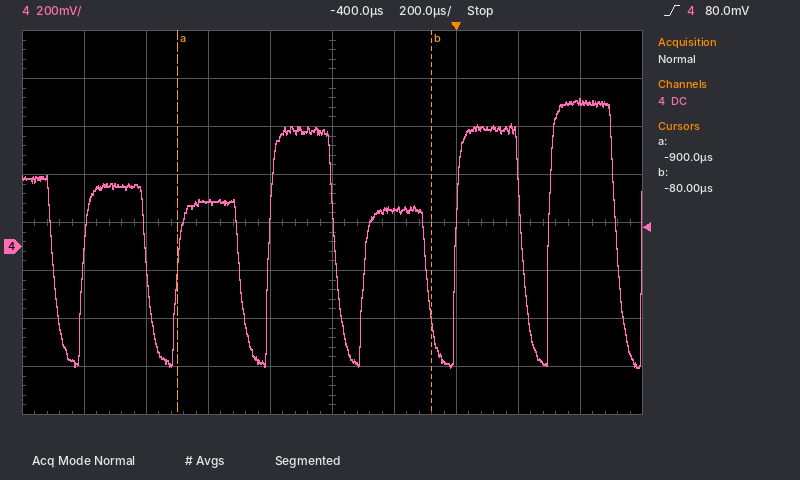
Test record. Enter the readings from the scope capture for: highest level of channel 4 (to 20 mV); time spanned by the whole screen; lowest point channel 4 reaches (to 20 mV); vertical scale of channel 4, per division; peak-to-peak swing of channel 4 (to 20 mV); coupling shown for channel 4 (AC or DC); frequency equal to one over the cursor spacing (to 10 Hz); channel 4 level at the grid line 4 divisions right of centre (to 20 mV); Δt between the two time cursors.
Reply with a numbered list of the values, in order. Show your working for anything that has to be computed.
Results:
1. 620 mV
2. 2 ms
3. -500 mV
4. 200 mV
5. 620 mV − (-500 mV) = 1.12 V
6. DC
7. 1 / 820 µs ≈ 1.22 kHz
8. 600 mV
9. -80 µs − (-900 µs) = 820 µs
